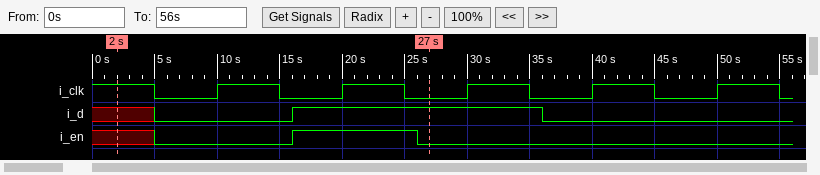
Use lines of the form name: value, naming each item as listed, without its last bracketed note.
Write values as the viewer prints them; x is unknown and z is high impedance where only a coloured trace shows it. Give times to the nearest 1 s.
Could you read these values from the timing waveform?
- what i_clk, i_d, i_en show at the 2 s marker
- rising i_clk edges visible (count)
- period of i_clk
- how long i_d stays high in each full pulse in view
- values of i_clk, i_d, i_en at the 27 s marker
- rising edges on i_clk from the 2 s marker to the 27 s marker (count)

what i_clk, i_d, i_en show at the 2 s marker: i_clk=1, i_d=x, i_en=x
rising i_clk edges visible: 5
period of i_clk: 10 s
how long i_d stays high in each full pulse in view: 20 s
values of i_clk, i_d, i_en at the 27 s marker: i_clk=0, i_d=1, i_en=0
rising edges on i_clk from the 2 s marker to the 27 s marker: 2
